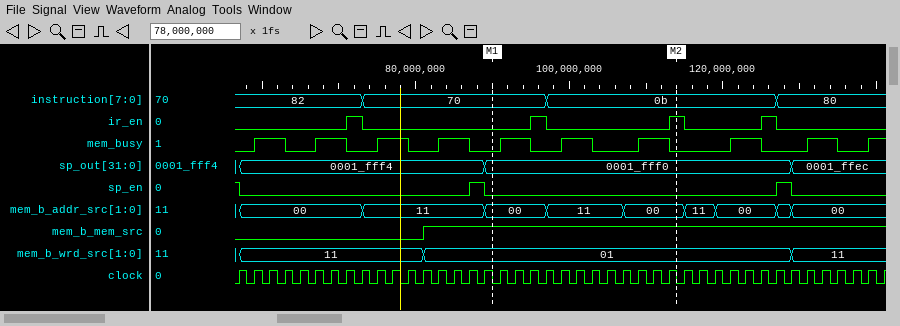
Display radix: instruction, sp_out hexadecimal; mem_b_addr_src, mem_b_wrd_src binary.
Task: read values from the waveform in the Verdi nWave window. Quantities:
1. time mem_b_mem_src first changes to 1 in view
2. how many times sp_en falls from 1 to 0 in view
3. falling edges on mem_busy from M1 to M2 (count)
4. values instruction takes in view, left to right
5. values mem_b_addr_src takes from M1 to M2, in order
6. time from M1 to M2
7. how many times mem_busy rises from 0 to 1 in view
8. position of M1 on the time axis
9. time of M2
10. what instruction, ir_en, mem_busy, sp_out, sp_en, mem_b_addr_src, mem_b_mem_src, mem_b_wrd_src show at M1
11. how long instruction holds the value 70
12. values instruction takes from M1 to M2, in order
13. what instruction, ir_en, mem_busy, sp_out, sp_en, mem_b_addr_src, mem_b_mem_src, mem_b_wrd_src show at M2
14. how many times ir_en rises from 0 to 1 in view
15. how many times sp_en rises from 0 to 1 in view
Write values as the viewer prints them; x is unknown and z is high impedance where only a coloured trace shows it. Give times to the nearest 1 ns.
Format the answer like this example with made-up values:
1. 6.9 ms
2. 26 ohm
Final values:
1. 81 ns
2. 3
3. 3
4. 82, 70, 0b, 80
5. 00, 11, 00
6. 24 ns
7. 10
8. 90 ns
9. 114 ns
10. instruction=70, ir_en=0, mem_busy=0, sp_out=0001_fff0, sp_en=0, mem_b_addr_src=00, mem_b_mem_src=1, mem_b_wrd_src=01
11. 24 ns
12. 70, 0b
13. instruction=0b, ir_en=1, mem_busy=0, sp_out=0001_fff0, sp_en=0, mem_b_addr_src=00, mem_b_mem_src=1, mem_b_wrd_src=01
14. 4
15. 2
